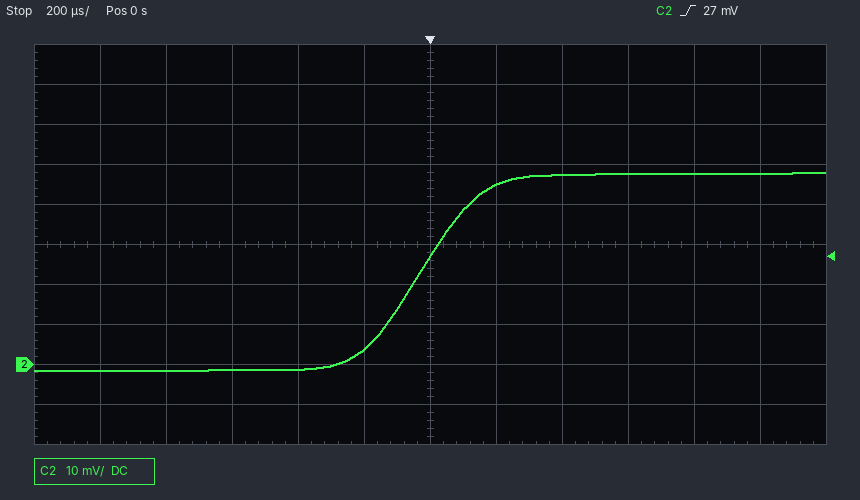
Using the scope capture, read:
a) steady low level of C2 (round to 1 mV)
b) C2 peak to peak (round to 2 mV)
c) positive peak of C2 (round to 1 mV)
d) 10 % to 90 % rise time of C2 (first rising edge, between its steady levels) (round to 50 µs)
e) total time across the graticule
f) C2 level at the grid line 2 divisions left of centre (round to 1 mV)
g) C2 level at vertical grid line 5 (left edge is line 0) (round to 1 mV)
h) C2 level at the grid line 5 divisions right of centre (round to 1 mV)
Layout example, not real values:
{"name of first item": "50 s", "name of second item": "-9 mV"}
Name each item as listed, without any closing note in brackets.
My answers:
{"steady low level of C2": "-1 mV", "C2 peak to peak": "50 mV", "positive peak of C2": "48 mV", "10 % to 90 % rise time of C2 (first rising edge, between its steady levels)": "350 µs", "total time across the graticule": "2.4 ms", "C2 level at the grid line 2 divisions left of centre": "-1 mV", "C2 level at vertical grid line 5 (left edge is line 0)": "4 mV", "C2 level at the grid line 5 divisions right of centre": "48 mV"}
